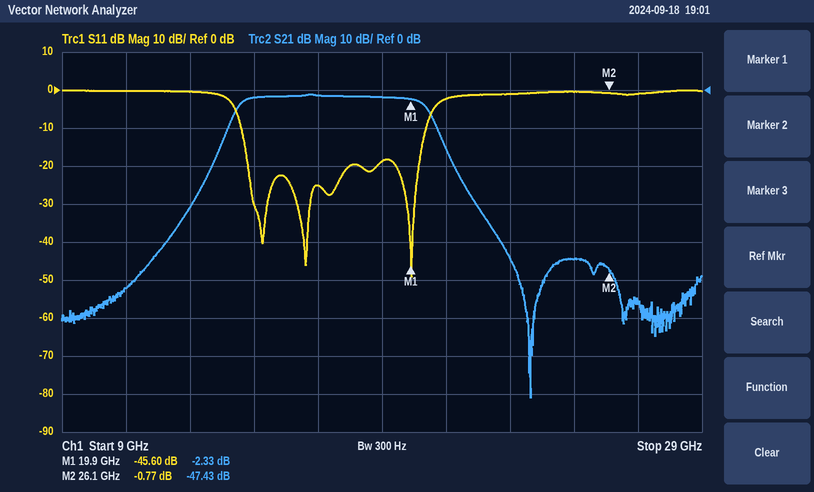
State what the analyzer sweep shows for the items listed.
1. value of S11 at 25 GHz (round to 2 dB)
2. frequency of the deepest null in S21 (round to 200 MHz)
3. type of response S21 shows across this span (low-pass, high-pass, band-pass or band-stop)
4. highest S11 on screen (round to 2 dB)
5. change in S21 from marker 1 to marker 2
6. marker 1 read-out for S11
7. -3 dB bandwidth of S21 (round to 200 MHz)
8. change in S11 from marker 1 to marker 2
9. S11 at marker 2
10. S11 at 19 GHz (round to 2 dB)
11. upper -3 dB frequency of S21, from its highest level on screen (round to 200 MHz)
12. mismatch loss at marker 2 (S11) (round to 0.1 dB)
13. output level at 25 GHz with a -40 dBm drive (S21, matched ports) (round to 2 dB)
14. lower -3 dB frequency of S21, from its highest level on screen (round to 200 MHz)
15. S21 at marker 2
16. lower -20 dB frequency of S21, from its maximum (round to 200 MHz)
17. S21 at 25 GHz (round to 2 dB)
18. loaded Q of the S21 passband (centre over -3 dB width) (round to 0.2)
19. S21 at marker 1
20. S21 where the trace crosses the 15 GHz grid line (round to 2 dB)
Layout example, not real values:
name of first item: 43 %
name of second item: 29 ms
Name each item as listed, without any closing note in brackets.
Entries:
value of S11 at 25 GHz: 0 dB
frequency of the deepest null in S21: 23.6 GHz
type of response S21 shows across this span: band-pass
highest S11 on screen: 0 dB
change in S21 from marker 1 to marker 2: -45.10 dB
marker 1 read-out for S11: -45.60 dB
-3 dB bandwidth of S21: 5.8 GHz
change in S11 from marker 1 to marker 2: 44.83 dB
S11 at marker 2: -0.77 dB
S11 at 19 GHz: -18 dB
upper -3 dB frequency of S21, from its highest level on screen: 20.4 GHz
mismatch loss at marker 2 (S11): 7.9 dB
output level at 25 GHz with a -40 dBm drive (S21, matched ports): -84 dBm
lower -3 dB frequency of S21, from its highest level on screen: 14.6 GHz
S21 at marker 2: -47.43 dB
lower -20 dB frequency of S21, from its maximum: 13.6 GHz
S21 at 25 GHz: -44 dB
loaded Q of the S21 passband (centre over -3 dB width): 3.0
S21 at marker 1: -2.33 dB
S21 where the trace crosses the 15 GHz grid line: -2 dB
